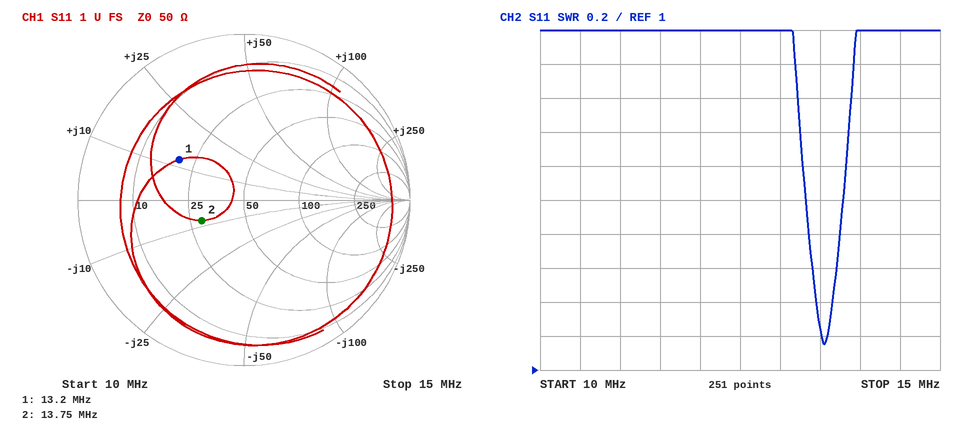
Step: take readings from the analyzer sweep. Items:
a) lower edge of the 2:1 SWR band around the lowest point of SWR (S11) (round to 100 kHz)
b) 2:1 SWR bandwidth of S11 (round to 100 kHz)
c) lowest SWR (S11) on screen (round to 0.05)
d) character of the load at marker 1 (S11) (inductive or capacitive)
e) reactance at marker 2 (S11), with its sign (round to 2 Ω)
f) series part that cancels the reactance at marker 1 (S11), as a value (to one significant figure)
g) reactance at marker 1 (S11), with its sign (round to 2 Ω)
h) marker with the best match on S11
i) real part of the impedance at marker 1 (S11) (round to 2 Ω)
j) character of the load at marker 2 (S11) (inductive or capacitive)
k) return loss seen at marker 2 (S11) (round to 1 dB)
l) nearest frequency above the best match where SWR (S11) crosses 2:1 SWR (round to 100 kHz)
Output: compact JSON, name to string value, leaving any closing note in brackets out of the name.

{"lower edge of the 2:1 SWR band around the lowest point of SWR (S11)": "13.3 MHz", "2:1 SWR bandwidth of S11": "500 kHz", "lowest SWR (S11) on screen": "1.15", "character of the load at marker 1 (S11)": "inductive", "reactance at marker 2 (S11), with its sign": "-8 Ω", "series part that cancels the reactance at marker 1 (S11), as a value": "1.0 nF", "reactance at marker 1 (S11), with its sign": "+12 Ω", "marker with the best match on S11": "marker 2", "real part of the impedance at marker 1 (S11)": "20 Ω", "character of the load at marker 2 (S11)": "capacitive", "return loss seen at marker 2 (S11)": "11 dB", "nearest frequency above the best match where SWR (S11) crosses 2:1 SWR": "13.8 MHz"}
